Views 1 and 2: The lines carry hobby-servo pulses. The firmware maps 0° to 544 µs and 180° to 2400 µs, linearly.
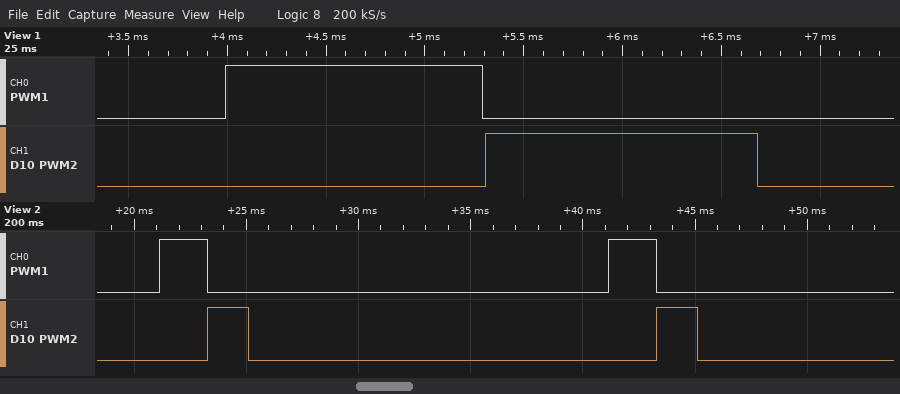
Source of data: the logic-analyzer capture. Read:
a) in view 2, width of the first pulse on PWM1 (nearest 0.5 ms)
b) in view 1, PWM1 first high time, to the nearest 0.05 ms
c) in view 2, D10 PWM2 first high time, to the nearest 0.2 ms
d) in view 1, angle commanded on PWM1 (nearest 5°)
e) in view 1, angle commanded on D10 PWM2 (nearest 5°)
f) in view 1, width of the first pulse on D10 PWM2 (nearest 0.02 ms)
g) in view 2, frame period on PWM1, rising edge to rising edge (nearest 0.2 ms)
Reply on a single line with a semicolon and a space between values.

2.0 ms; 1.30 ms; 1.8 ms; 75°; 80°; 1.38 ms; 20.0 ms
